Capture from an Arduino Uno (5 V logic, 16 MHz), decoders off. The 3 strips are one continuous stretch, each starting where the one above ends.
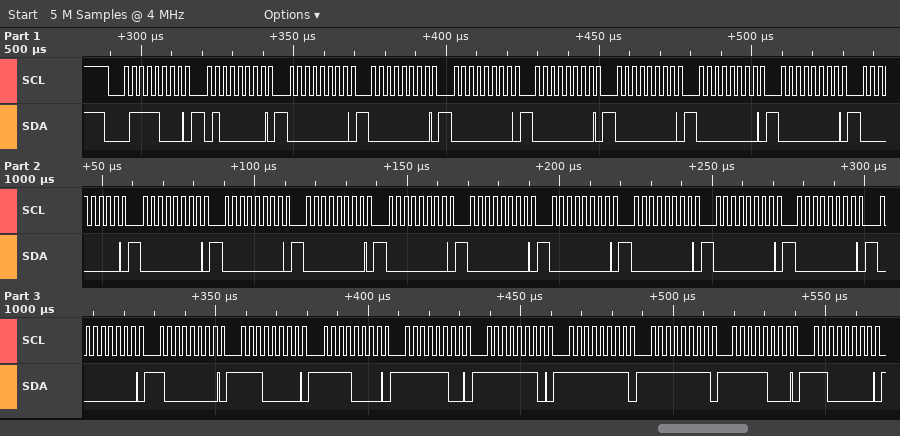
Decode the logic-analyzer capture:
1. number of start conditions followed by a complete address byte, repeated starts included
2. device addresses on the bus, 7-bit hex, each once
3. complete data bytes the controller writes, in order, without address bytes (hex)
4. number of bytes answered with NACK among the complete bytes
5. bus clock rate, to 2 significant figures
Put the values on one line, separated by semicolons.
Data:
1; 0x3C; 40 00 00 00 00 00 00 00 00 00 00 00 00 00 00 00 00 00 00 80 E0 F0 FC FE FF FF F8 C0; 0; 400 kHz
